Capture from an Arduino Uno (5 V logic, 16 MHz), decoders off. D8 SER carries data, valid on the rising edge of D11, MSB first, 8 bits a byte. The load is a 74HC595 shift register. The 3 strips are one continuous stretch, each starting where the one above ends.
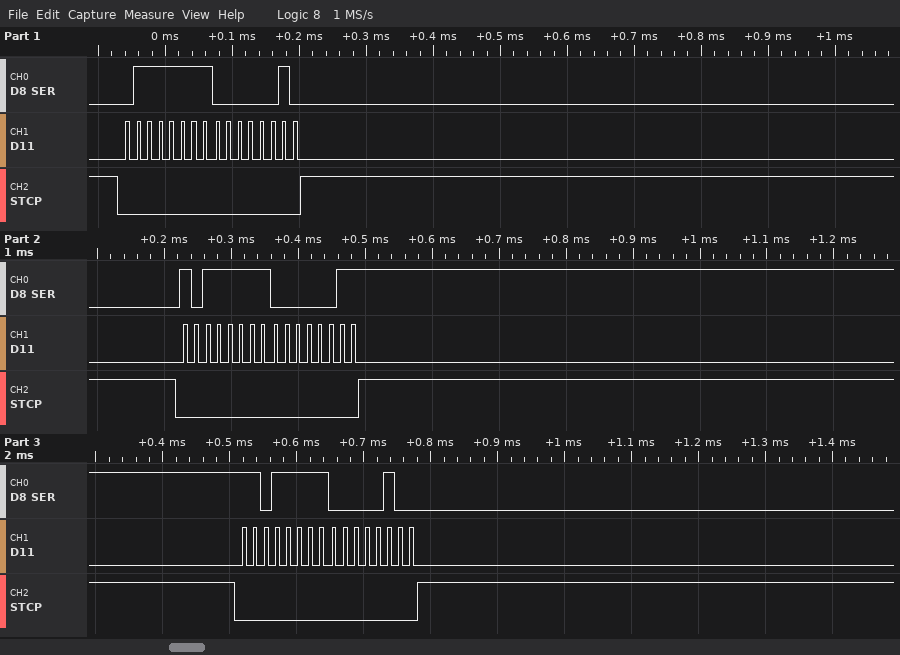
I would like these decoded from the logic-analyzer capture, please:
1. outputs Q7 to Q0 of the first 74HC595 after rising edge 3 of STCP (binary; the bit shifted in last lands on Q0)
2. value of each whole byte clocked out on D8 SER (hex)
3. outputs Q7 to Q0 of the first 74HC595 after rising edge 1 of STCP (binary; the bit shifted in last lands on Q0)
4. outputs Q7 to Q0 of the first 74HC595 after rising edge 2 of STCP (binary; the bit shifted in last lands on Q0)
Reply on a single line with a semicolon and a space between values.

00000100; 7F 02 BF 03 DF 04; 00000010; 00000011
